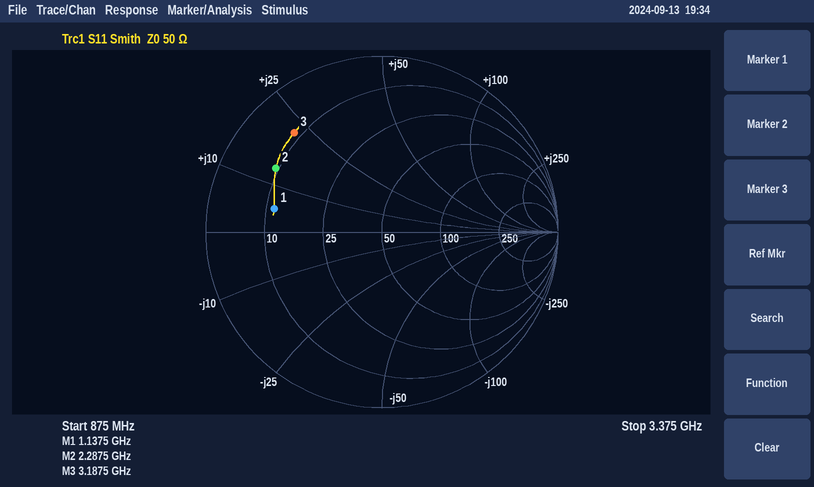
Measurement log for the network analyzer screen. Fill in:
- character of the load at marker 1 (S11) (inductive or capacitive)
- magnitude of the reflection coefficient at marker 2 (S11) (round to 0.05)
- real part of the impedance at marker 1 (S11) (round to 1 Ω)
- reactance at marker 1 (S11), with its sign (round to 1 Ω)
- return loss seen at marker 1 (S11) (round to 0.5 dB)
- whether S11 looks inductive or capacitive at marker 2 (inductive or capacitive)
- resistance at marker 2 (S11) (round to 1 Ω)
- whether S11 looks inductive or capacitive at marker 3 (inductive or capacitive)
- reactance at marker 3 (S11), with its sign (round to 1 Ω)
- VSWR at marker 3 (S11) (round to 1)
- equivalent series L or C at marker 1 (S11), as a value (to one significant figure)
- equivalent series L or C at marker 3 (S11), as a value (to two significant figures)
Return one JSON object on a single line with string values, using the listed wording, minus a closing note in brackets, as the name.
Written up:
{"character of the load at marker 1 (S11)": "inductive", "magnitude of the reflection coefficient at marker 2 (S11)": "0.70", "real part of the impedance at marker 1 (S11)": "12 Ω", "reactance at marker 1 (S11), with its sign": "+5 Ω", "return loss seen at marker 1 (S11)": "4.0 dB", "whether S11 looks inductive or capacitive at marker 2": "inductive", "resistance at marker 2 (S11)": "9 Ω", "whether S11 looks inductive or capacitive at marker 3": "inductive", "reactance at marker 3 (S11), with its sign": "+22 Ω", "VSWR at marker 3 (S11)": "7", "equivalent series L or C at marker 1 (S11), as a value": "700 pH", "equivalent series L or C at marker 3 (S11), as a value": "1.1 nH"}
